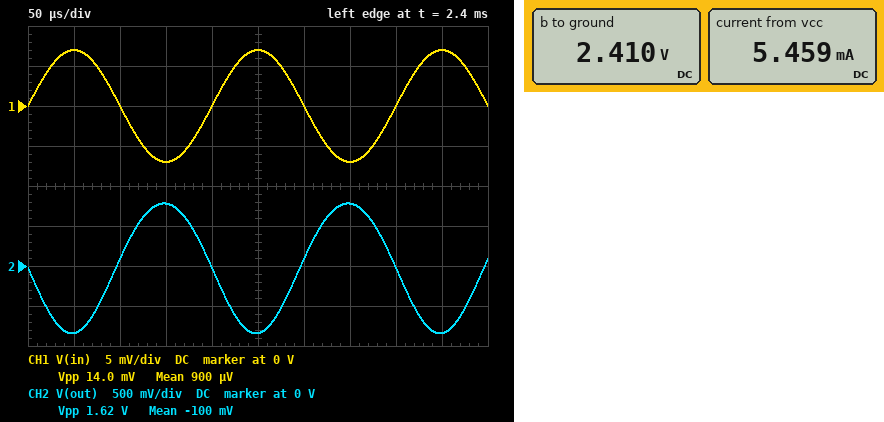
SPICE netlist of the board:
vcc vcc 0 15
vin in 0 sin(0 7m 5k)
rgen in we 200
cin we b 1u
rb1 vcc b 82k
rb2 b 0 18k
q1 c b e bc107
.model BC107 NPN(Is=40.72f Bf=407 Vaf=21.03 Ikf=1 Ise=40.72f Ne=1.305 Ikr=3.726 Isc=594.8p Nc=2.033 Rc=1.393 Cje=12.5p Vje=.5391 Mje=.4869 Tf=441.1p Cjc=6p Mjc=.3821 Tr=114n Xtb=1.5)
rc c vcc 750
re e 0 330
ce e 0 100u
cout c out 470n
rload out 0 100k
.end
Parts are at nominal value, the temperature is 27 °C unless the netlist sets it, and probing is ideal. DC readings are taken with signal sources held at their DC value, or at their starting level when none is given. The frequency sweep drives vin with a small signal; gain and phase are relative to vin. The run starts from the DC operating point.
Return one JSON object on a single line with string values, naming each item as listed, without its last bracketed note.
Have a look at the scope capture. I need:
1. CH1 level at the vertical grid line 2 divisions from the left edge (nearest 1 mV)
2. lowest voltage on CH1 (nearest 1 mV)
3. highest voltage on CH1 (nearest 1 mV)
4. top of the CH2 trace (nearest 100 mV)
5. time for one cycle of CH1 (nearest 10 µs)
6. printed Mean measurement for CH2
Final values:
{"CH1 level at the vertical grid line 2 divisions from the left edge": "0 V", "lowest voltage on CH1": "-7 mV", "highest voltage on CH1": "7 mV", "top of the CH2 trace": "800 mV", "time for one cycle of CH1": "200 µs", "printed Mean measurement for CH2": "-100 mV"}
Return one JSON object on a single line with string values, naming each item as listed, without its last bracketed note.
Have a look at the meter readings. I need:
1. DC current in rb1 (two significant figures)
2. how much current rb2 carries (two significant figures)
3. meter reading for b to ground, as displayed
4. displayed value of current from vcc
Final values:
{"DC current in rb1": "150 µA", "how much current rb2 carries": "130 µA", "meter reading for b to ground, as displayed": "2.410 V", "displayed value of current from vcc": "5.459 mA"}
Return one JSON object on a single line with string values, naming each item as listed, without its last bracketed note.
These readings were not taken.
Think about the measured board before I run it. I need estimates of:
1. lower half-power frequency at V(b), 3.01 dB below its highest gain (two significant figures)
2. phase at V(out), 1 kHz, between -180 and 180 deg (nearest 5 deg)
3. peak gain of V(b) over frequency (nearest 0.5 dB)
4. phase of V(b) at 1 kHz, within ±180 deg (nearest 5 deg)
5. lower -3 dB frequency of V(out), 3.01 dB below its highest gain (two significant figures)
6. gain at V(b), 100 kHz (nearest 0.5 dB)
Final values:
{"lower half-power frequency at V(b), 3.01 dB below its highest gain": "15 Hz", "phase at V(out), 1 kHz, between -180 and 180 deg": "-160 deg", "peak gain of V(b) over frequency": "-1.0 dB", "phase of V(b) at 1 kHz, within ±180 deg": "5 deg", "lower -3 dB frequency of V(out), 3.01 dB below its highest gain": "350 Hz", "gain at V(b), 100 kHz": "-1.0 dB"}
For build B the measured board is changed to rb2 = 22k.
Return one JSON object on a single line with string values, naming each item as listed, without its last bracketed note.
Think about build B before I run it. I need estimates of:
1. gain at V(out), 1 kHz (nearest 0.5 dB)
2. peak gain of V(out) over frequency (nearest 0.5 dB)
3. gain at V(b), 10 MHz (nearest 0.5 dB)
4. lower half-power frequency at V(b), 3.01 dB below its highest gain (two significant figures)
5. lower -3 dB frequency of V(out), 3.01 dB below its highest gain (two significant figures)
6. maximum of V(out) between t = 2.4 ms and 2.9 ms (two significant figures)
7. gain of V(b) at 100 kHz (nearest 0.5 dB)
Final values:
{"gain at V(out), 1 kHz": "42.0 dB", "peak gain of V(out) over frequency": "42.5 dB", "gain at V(b), 10 MHz": "-16.0 dB", "lower half-power frequency at V(b), 3.01 dB below its highest gain": "12 Hz", "lower -3 dB frequency of V(out), 3.01 dB below its highest gain": "400 Hz", "maximum of V(out) between t = 2.4 ms and 2.9 ms": "890 mV", "gain of V(b) at 100 kHz": "-1.5 dB"}
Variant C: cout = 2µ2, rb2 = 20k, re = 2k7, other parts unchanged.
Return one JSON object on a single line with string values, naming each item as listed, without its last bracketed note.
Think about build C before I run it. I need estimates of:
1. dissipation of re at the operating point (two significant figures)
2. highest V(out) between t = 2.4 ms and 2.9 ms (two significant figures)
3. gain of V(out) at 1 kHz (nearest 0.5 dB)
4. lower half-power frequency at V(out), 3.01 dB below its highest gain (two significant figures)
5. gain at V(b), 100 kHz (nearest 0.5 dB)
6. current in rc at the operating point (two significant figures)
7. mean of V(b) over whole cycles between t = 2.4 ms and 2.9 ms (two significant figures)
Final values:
{"dissipation of re at the operating point": "1.9 mW", "highest V(out) between t = 2.4 ms and 2.9 ms": "150 mV", "gain of V(out) at 1 kHz": "27.0 dB", "lower half-power frequency at V(out), 3.01 dB below its highest gain": "72 Hz", "gain at V(b), 100 kHz": "-0.5 dB", "current in rc at the operating point": "840 µA", "mean of V(b) over whole cycles between t = 2.4 ms and 2.9 ms": "2.9 V"}
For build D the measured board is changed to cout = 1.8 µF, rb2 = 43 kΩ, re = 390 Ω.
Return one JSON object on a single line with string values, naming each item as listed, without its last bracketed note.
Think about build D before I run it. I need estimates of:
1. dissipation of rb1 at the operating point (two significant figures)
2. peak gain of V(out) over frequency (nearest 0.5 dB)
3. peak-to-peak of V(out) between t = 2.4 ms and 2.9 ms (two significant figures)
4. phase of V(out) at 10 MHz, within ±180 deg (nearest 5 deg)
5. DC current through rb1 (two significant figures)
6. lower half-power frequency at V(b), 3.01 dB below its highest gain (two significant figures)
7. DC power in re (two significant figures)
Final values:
{"dissipation of rb1 at the operating point": "1.4 mW", "peak gain of V(out) over frequency": "44.0 dB", "peak-to-peak of V(out) between t = 2.4 ms and 2.9 ms": "2.2 V", "phase of V(out) at 10 MHz, within ±180 deg": "95 deg", "DC current through rb1": "130 µA", "lower half-power frequency at V(b), 3.01 dB below its highest gain": "7.6 Hz", "DC power in re": "31 mW"}
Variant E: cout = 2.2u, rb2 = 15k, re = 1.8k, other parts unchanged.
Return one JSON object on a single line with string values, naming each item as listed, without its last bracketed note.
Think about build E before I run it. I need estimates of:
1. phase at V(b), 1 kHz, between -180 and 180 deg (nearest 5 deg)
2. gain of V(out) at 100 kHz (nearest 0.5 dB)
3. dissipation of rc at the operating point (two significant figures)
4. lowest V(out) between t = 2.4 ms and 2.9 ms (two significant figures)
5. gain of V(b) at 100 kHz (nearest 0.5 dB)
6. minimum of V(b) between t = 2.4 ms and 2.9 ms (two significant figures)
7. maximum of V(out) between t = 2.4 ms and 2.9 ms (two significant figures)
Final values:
{"phase at V(b), 1 kHz, between -180 and 180 deg": "0 deg", "gain of V(out) at 100 kHz": "28.0 dB", "dissipation of rc at the operating point": "640 µW", "lowest V(out) between t = 2.4 ms and 2.9 ms": "-190 mV", "gain of V(b) at 100 kHz": "-0.5 dB", "minimum of V(b) between t = 2.4 ms and 2.9 ms": "2.3 V", "maximum of V(out) between t = 2.4 ms and 2.9 ms": "160 mV"}
